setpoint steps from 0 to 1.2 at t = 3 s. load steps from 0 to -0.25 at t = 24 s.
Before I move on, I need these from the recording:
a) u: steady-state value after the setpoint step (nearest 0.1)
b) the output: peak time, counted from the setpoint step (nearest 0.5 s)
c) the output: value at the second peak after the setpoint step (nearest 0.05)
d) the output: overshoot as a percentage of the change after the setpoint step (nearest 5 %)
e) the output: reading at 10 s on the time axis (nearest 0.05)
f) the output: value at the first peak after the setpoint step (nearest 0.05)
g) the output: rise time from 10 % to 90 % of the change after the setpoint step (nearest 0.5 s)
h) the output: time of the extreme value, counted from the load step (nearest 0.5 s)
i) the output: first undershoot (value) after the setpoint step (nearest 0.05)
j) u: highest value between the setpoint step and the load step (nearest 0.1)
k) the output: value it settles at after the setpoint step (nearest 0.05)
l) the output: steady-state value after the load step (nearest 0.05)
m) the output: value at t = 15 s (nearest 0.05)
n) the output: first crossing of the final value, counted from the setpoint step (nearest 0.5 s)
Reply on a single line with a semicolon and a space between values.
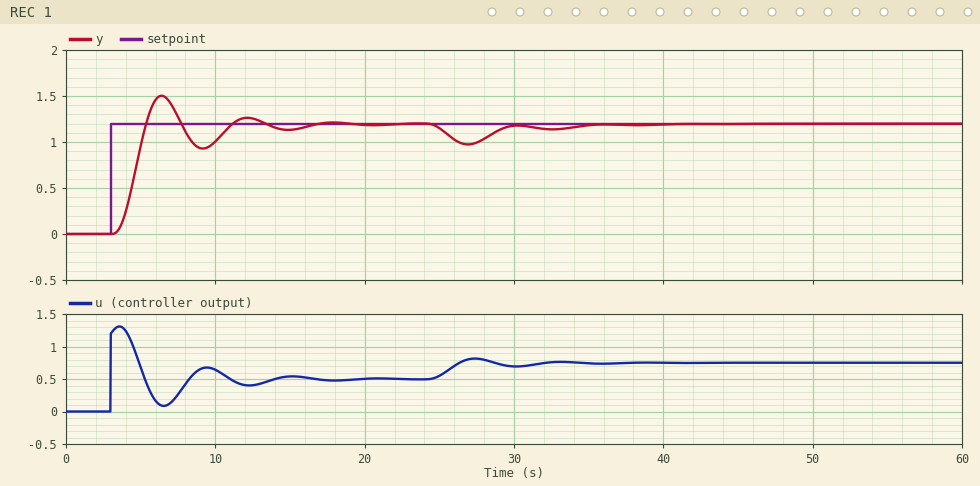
0.5; 3.5 s; 1.25; 25 %; 1.00; 1.50; 1.5 s; 3.0 s; 0.95; 1.3; 1.20; 1.20; 1.15; 2.5 s
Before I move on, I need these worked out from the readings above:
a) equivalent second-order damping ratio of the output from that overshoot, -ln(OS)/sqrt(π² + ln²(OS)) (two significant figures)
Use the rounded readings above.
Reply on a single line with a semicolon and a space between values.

0.40
